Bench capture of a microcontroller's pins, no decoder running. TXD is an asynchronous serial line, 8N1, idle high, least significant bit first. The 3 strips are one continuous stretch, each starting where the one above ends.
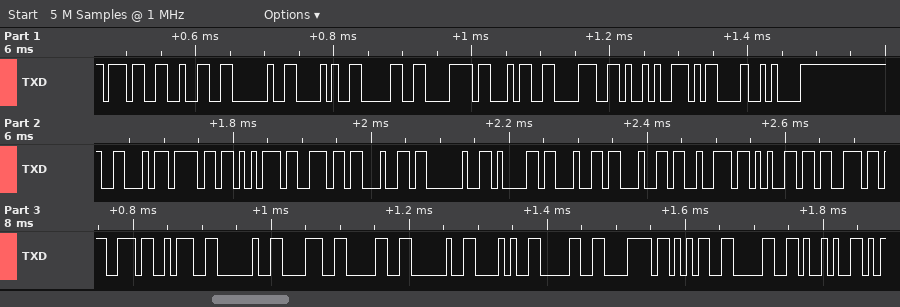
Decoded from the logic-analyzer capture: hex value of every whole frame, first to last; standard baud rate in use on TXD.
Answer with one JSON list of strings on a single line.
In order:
["37 32 20 28 30 78 34 38 29 0D 0A 46 6F 75 6E 64 20 61 64 64 72 65 73 73 3A 20 38 30 20 28 30 78 35 30 29", "115200 baud"]
